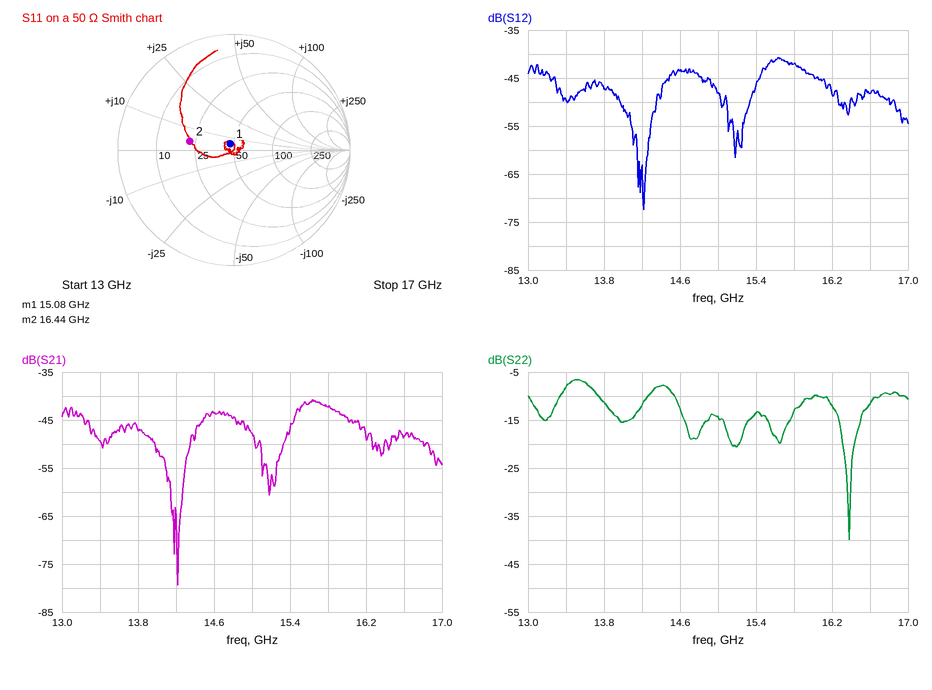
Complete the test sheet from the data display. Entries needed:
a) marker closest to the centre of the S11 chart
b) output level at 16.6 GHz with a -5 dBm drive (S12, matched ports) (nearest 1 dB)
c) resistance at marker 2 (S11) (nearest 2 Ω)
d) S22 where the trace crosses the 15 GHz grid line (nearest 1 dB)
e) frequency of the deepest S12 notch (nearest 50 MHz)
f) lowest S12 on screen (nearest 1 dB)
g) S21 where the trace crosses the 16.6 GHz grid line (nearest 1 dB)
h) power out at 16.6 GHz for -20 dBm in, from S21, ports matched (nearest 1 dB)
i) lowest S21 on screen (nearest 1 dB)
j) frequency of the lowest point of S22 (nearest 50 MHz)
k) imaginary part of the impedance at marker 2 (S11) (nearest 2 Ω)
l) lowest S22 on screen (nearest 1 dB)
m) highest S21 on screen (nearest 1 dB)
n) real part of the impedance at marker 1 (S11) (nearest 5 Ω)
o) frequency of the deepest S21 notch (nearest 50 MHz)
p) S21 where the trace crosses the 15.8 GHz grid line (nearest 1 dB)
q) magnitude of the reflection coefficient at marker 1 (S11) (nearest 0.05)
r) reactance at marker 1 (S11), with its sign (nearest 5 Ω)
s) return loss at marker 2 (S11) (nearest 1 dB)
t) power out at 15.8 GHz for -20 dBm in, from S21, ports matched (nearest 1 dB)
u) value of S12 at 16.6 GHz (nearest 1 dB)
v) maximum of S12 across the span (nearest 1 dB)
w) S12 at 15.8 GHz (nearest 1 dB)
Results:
marker 1
-53 dBm
22 Ω
-14 dB
14.20 GHz
-72 dB
-48 dB
-68 dBm
-79 dB
16.40 GHz
+4 Ω
-40 dB
-41 dB
45 Ω
14.20 GHz
-42 dB
0.05
+5 Ω
8 dB
-62 dBm
-48 dB
-41 dB
-42 dB
